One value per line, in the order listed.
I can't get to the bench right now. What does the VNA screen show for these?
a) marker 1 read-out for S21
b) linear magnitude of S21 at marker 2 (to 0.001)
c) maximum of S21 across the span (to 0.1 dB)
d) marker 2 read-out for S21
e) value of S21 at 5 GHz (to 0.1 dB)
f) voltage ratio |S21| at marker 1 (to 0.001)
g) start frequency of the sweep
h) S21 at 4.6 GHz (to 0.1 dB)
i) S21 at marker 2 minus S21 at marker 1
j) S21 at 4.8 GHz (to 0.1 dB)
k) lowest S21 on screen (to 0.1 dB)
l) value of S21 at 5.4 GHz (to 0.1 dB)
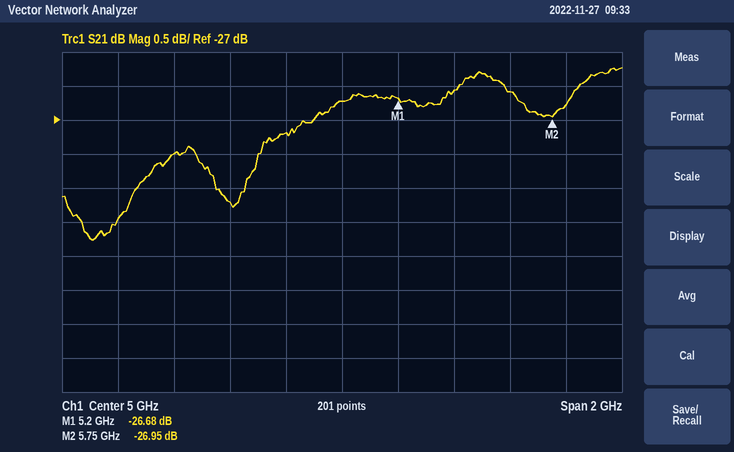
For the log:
-26.68 dB
0.045
-26.2 dB
-26.95 dB
-26.7 dB
0.046
4 GHz
-28.2 dB
-0.27 dB
-27.2 dB
-28.8 dB
-26.6 dB
